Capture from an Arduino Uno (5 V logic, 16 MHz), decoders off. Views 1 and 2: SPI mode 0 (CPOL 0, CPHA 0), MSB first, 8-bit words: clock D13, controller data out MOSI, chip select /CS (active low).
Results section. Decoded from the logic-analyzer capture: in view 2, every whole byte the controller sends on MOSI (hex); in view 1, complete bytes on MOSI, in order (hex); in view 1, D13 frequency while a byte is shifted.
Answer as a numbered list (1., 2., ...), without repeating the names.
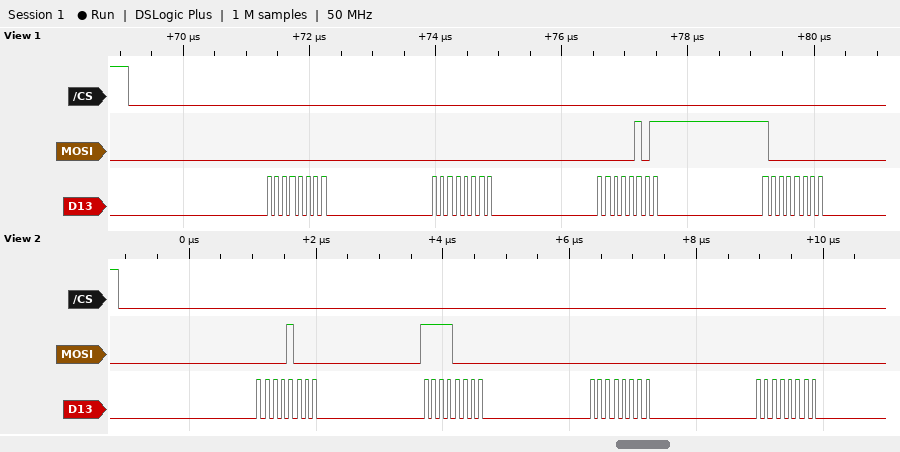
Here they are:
1. 0x08 0xF0 0x00 0x00
2. 00 00 05 80
3. 8 MHz
